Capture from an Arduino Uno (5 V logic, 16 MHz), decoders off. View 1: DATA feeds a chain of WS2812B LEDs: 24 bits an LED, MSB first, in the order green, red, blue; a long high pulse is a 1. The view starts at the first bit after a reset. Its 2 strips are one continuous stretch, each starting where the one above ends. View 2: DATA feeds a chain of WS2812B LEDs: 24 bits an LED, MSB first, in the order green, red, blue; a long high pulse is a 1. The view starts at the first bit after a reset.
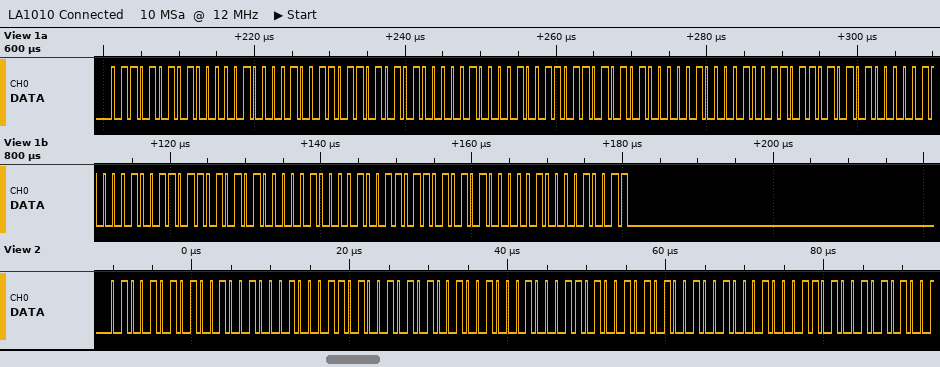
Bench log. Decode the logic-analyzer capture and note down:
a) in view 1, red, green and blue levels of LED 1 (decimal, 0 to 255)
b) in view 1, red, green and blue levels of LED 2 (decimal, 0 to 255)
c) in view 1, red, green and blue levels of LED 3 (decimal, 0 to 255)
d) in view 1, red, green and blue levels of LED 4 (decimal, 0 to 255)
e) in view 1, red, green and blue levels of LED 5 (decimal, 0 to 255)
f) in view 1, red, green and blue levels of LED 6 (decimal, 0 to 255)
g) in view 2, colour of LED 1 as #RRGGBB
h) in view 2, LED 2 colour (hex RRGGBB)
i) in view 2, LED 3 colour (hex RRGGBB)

130, 106, 19
130, 106, 19
130, 106, 19
130, 106, 19
130, 106, 19
130, 106, 19
#924A23
#924A23
#924A23
